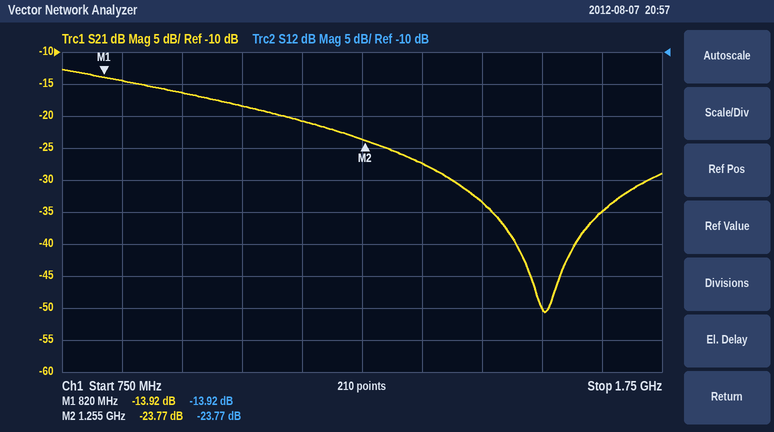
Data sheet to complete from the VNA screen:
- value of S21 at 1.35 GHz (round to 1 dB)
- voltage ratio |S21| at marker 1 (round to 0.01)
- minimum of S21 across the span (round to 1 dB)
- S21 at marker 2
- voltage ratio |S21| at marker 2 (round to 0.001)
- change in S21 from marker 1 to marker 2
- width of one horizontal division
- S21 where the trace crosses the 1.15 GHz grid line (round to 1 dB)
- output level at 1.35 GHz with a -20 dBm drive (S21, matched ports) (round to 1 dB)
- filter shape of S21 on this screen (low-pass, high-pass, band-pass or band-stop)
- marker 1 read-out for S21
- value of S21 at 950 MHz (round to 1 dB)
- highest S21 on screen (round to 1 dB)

-27 dB
0.20
-51 dB
-23.77 dB
0.065
-9.85 dB
100 MHz
-21 dB
-47 dBm
low-pass
-13.92 dB
-16 dB
-13 dB
